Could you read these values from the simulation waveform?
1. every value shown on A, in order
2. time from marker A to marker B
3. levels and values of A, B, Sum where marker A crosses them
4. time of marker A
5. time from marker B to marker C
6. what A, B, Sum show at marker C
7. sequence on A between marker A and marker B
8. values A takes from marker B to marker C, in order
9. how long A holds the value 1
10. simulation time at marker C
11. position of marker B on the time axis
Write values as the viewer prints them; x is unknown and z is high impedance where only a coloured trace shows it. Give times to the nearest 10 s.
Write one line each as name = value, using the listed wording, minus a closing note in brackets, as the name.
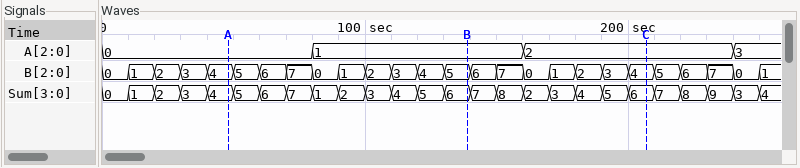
every value shown on A, in order = 0, 1, 2, 3
time from marker A to marker B = 90 s
levels and values of A, B, Sum where marker A crosses them = A=0, B=4, Sum=4
time of marker A = 50 s
time from marker B to marker C = 70 s
what A, B, Sum show at marker C = A=2, B=4, Sum=6
sequence on A between marker A and marker B = 0, 1
values A takes from marker B to marker C, in order = 1, 2
how long A holds the value 1 = 80 s
simulation time at marker C = 210 s
position of marker B on the time axis = 140 s
